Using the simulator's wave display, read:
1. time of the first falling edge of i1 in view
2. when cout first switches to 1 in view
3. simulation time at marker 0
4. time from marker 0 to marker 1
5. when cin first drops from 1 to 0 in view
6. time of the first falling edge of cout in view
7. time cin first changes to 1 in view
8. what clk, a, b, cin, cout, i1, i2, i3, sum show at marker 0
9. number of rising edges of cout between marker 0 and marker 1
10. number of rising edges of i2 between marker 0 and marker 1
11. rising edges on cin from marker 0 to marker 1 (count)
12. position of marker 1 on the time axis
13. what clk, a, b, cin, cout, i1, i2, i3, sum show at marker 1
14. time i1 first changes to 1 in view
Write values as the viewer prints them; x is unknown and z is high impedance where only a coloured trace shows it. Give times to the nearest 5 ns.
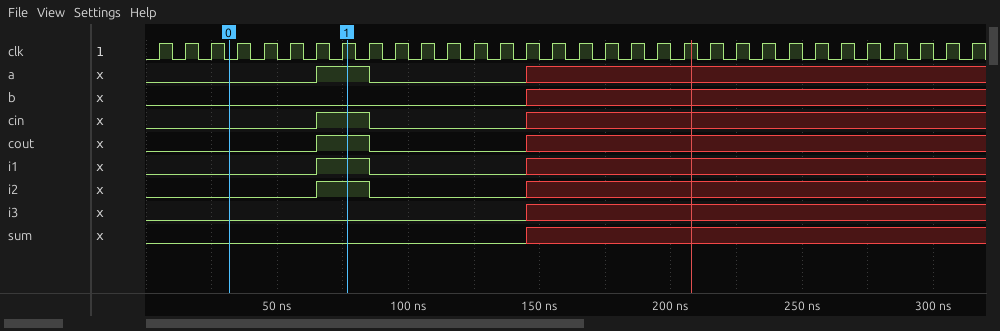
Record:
85 ns
65 ns
30 ns
45 ns
85 ns
85 ns
65 ns
clk=0, a=0, b=0, cin=0, cout=0, i1=0, i2=0, i3=0, sum=0
1
1
1
75 ns
clk=1, a=1, b=0, cin=1, cout=1, i1=1, i2=1, i3=0, sum=0
65 ns
